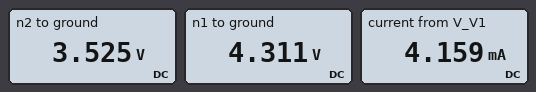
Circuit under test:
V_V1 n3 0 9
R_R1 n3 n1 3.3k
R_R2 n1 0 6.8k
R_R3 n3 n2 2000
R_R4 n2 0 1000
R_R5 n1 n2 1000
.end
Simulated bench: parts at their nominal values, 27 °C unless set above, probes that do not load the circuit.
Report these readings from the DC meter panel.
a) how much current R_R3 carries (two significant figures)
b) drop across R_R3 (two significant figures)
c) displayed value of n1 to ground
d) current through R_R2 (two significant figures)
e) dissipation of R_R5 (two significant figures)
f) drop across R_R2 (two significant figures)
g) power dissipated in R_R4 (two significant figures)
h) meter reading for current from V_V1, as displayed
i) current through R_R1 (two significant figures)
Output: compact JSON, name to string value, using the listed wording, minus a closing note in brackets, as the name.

{"how much current R_R3 carries": "2.7 mA", "drop across R_R3": "5.5 V", "displayed value of n1 to ground": "4.311 V", "current through R_R2": "630 µA", "dissipation of R_R5": "620 µW", "drop across R_R2": "4.3 V", "power dissipated in R_R4": "12 mW", "meter reading for current from V_V1, as displayed": "4.159 mA", "current through R_R1": "1.4 mA"}
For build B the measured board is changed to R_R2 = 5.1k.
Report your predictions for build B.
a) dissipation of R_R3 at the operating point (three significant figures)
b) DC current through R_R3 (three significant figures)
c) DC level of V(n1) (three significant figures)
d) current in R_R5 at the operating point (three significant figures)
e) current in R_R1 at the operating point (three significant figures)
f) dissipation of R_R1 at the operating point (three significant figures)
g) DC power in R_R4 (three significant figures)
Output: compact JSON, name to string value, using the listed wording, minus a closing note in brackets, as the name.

{"dissipation of R_R3 at the operating point": "15.4 mW", "DC current through R_R3": "2.78 mA", "DC level of V(n1)": "4.12 V", "current in R_R5 at the operating point": "671 µA", "current in R_R1 at the operating point": "1.48 mA", "dissipation of R_R1 at the operating point": "7.22 mW", "DC power in R_R4": "11.9 mW"}
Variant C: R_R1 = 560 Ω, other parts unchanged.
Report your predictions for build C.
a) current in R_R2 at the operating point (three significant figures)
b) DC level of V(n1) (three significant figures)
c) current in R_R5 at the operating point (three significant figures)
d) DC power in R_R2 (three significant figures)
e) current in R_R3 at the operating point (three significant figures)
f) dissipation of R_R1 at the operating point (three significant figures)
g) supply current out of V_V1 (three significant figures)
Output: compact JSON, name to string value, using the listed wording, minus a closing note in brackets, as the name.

{"current in R_R2 at the operating point": "1.04 mA", "DC level of V(n1)": "7.06 V", "current in R_R5 at the operating point": "2.43 mA", "DC power in R_R2": "7.32 mW", "current in R_R3 at the operating point": "2.19 mA", "dissipation of R_R1 at the operating point": "6.75 mW", "supply current out of V_V1": "5.66 mA"}
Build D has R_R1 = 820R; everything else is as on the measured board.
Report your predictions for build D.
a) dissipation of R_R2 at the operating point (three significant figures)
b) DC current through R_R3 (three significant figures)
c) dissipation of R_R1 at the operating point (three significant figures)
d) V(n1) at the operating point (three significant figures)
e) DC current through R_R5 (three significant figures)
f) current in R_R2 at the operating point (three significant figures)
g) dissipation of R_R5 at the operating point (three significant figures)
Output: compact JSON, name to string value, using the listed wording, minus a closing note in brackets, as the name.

{"dissipation of R_R2 at the operating point": "6.21 mW", "DC current through R_R3": "2.30 mA", "dissipation of R_R1 at the operating point": "7.64 mW", "V(n1) at the operating point": "6.50 V", "DC current through R_R5": "2.10 mA", "current in R_R2 at the operating point": "955 µA", "dissipation of R_R5 at the operating point": "4.40 mW"}
